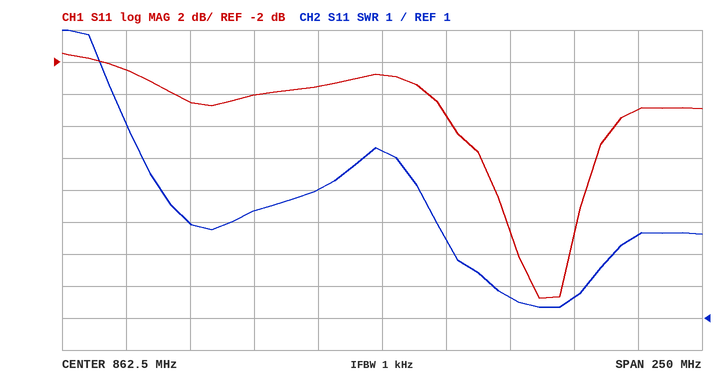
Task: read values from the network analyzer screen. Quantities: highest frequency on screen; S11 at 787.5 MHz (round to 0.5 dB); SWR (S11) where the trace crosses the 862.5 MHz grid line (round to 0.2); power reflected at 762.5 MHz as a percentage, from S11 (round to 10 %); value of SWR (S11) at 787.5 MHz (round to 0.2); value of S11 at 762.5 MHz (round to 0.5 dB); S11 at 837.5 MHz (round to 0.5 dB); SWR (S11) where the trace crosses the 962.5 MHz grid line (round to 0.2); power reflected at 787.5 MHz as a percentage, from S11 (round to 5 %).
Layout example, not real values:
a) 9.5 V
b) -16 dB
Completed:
a) 987.5 MHz
b) -4.5 dB
c) 6.2
d) 60 %
e) 4.0
f) -2.5 dB
g) -3.5 dB
h) 3.6
i) 35 %
